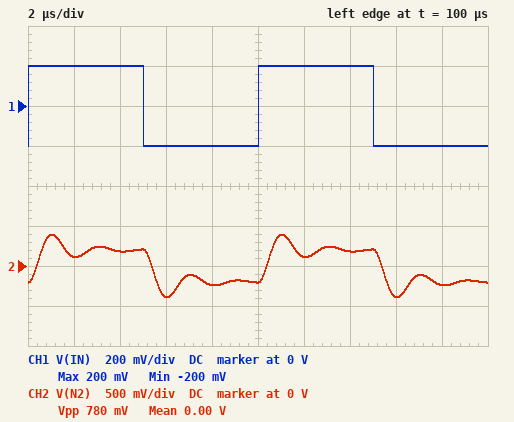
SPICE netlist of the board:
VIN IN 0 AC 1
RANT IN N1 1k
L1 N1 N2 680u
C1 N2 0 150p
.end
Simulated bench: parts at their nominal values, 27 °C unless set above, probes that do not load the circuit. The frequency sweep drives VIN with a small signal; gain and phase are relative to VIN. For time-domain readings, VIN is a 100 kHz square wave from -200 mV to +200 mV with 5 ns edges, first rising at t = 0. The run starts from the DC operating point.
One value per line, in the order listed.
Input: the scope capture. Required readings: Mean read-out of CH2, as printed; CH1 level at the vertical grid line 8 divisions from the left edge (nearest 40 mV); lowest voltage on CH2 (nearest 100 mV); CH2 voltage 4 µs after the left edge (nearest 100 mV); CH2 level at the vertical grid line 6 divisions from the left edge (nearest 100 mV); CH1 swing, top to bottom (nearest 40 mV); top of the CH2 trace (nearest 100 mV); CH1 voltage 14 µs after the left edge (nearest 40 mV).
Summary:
0.00 V
-200 mV
-400 mV
200 mV
100 mV
400 mV
400 mV
200 mV
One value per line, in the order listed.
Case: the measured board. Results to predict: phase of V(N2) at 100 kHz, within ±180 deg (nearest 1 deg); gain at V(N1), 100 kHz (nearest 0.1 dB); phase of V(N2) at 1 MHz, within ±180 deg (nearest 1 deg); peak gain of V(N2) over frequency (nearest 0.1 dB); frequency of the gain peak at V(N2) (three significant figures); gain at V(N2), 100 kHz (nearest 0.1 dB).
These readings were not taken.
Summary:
-6 deg
0 dB
-163 deg
6.8 dB
470 kHz
0.3 dB
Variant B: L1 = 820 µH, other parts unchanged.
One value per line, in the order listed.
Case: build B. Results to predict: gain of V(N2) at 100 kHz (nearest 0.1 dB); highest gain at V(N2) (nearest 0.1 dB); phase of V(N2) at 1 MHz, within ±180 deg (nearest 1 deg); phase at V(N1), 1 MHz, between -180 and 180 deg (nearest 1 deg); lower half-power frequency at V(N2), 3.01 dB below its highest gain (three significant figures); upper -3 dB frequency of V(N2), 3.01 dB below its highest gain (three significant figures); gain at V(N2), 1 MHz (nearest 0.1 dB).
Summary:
0.4 dB
7.6 dB
-166 deg
14 deg
318 kHz
523 kHz
-12.0 dB
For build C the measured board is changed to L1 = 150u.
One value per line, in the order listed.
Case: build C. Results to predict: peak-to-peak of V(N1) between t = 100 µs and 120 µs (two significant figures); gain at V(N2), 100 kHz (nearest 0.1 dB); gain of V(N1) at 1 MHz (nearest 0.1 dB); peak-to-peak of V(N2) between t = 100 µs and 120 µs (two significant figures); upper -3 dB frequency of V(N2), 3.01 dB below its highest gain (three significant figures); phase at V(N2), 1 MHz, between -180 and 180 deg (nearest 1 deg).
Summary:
470 mV
0 dB
-18.6 dB
530 mV
1.24 MHz
-83 deg
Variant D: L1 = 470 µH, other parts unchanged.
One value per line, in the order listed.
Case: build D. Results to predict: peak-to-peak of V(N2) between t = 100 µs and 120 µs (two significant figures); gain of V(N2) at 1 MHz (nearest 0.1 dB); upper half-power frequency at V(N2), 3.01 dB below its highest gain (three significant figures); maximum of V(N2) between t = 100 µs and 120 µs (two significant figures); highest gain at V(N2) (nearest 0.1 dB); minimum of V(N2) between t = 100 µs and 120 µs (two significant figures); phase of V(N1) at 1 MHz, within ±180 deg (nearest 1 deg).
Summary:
720 mV
-6.1 dB
705 kHz
360 mV
5.3 dB
-360 mV
28 deg
